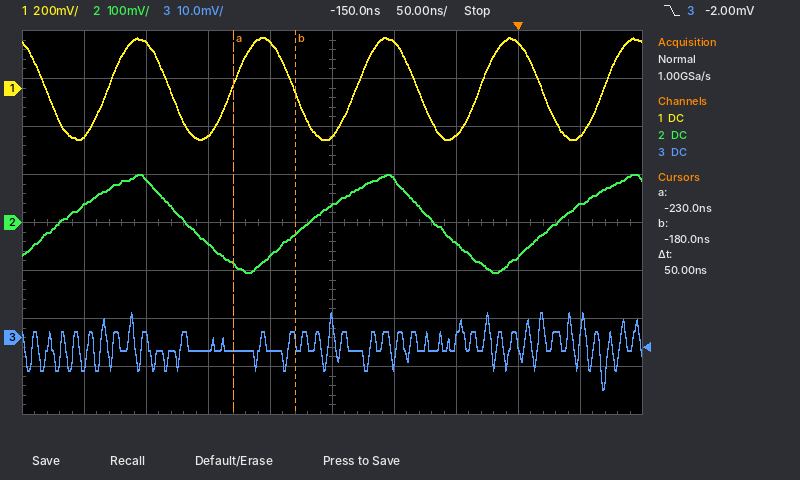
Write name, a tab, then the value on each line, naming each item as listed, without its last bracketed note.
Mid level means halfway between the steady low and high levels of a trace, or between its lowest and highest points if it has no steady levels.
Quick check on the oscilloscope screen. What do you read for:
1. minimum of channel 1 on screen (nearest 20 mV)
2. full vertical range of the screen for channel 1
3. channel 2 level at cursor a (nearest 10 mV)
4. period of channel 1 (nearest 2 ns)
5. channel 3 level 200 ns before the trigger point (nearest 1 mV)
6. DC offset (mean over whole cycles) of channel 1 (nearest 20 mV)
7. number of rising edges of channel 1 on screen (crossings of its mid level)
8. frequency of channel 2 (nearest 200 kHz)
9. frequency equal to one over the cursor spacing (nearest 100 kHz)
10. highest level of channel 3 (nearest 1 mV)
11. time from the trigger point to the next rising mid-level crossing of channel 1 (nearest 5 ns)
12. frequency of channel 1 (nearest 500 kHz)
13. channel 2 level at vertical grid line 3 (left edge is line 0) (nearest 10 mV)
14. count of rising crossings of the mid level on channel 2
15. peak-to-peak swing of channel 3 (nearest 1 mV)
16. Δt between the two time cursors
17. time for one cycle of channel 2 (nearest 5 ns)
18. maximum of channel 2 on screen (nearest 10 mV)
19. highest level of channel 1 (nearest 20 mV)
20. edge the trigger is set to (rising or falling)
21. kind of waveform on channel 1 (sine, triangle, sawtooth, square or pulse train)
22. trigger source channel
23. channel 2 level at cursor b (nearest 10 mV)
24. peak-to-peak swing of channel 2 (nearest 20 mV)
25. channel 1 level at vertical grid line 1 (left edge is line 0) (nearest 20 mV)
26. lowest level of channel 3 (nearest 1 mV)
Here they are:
minimum of channel 1 on screen	-220 mV
full vertical range of the screen for channel 1	1.6 V
channel 2 level at cursor a	-90 mV
period of channel 1	100 ns
channel 3 level 200 ns before the trigger point	-3 mV
DC offset (mean over whole cycles) of channel 1	0 mV
number of rising edges of channel 1 on screen	5
frequency of channel 2	5.0 MHz
frequency equal to one over the cursor spacing	20.0 MHz
highest level of channel 3	5 mV
time from the trigger point to the next rising mid-level crossing of channel 1	70 ns
frequency of channel 1	10.0 MHz
channel 2 level at vertical grid line 3 (left edge is line 0)	-40 mV
count of rising crossings of the mid level on channel 2	3
peak-to-peak swing of channel 3	16 mV
Δt between the two time cursors	50 ns
time for one cycle of channel 2	200 ns
maximum of channel 2 on screen	100 mV
highest level of channel 1	220 mV
edge the trigger is set to	falling
kind of waveform on channel 1	sine
trigger source channel	channel 3
channel 2 level at cursor b	-20 mV
peak-to-peak swing of channel 2	200 mV
channel 1 level at vertical grid line 1 (left edge is line 0)	-200 mV
lowest level of channel 3	-11 mV
